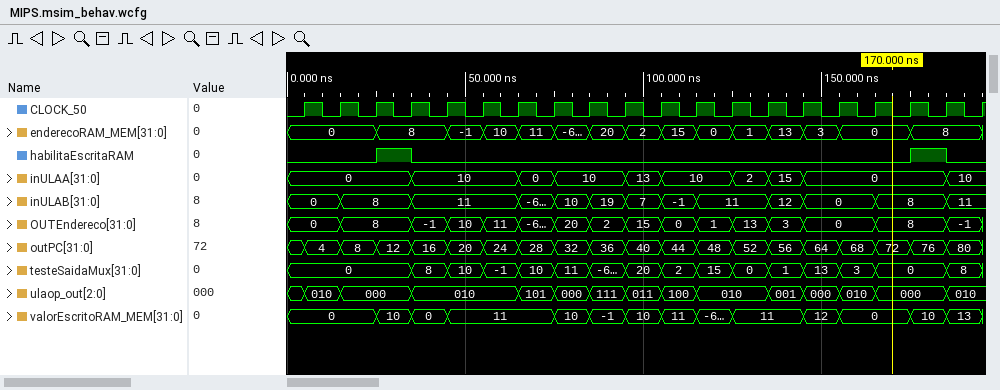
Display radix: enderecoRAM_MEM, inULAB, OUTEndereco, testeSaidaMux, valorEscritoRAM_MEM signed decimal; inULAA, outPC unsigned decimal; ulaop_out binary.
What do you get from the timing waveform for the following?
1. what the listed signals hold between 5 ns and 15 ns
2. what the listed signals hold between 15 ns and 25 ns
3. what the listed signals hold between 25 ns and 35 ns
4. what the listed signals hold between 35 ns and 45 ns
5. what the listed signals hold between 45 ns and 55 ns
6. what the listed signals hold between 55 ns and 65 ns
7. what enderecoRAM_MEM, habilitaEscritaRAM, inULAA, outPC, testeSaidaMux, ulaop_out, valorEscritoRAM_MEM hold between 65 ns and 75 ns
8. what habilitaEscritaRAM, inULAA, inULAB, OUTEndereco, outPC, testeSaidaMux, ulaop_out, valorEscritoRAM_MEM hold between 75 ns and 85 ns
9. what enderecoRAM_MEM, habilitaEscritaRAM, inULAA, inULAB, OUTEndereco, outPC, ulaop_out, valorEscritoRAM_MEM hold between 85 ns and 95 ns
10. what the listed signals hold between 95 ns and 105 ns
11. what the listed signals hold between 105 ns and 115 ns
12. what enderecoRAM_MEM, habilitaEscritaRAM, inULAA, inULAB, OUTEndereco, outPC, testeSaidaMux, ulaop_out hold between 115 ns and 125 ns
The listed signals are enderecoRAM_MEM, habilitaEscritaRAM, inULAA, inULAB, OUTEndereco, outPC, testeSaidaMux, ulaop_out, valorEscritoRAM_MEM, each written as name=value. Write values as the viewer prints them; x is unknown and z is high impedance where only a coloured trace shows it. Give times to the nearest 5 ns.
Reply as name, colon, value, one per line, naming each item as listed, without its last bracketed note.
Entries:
what the listed signals hold between 5 ns and 15 ns: enderecoRAM_MEM=0, habilitaEscritaRAM=0, inULAA=0, inULAB=0, OUTEndereco=0, outPC=4, testeSaidaMux=0, ulaop_out=010, valorEscritoRAM_MEM=0
what the listed signals hold between 15 ns and 25 ns: enderecoRAM_MEM=0, habilitaEscritaRAM=0, inULAA=0, inULAB=8, OUTEndereco=8, outPC=8, testeSaidaMux=0, ulaop_out=000, valorEscritoRAM_MEM=0
what the listed signals hold between 25 ns and 35 ns: enderecoRAM_MEM=8, habilitaEscritaRAM=1, inULAA=0, inULAB=8, OUTEndereco=8, outPC=12, testeSaidaMux=0, ulaop_out=000, valorEscritoRAM_MEM=10
what the listed signals hold between 35 ns and 45 ns: enderecoRAM_MEM=8, habilitaEscritaRAM=0, inULAA=10, inULAB=11, OUTEndereco=-1, outPC=16, testeSaidaMux=8, ulaop_out=010, valorEscritoRAM_MEM=0
what the listed signals hold between 45 ns and 55 ns: enderecoRAM_MEM=-1, habilitaEscritaRAM=0, inULAA=10, inULAB=11, OUTEndereco=10, outPC=20, testeSaidaMux=10, ulaop_out=010, valorEscritoRAM_MEM=11
what the listed signals hold between 55 ns and 65 ns: enderecoRAM_MEM=10, habilitaEscritaRAM=0, inULAA=10, inULAB=11, OUTEndereco=11, outPC=24, testeSaidaMux=-1, ulaop_out=010, valorEscritoRAM_MEM=11
what enderecoRAM_MEM, habilitaEscritaRAM, inULAA, outPC, testeSaidaMux, ulaop_out, valorEscritoRAM_MEM hold between 65 ns and 75 ns: enderecoRAM_MEM=11, habilitaEscritaRAM=0, inULAA=0, outPC=28, testeSaidaMux=10, ulaop_out=101, valorEscritoRAM_MEM=11
what habilitaEscritaRAM, inULAA, inULAB, OUTEndereco, outPC, testeSaidaMux, ulaop_out, valorEscritoRAM_MEM hold between 75 ns and 85 ns: habilitaEscritaRAM=0, inULAA=10, inULAB=10, OUTEndereco=20, outPC=32, testeSaidaMux=11, ulaop_out=000, valorEscritoRAM_MEM=10
what enderecoRAM_MEM, habilitaEscritaRAM, inULAA, inULAB, OUTEndereco, outPC, ulaop_out, valorEscritoRAM_MEM hold between 85 ns and 95 ns: enderecoRAM_MEM=20, habilitaEscritaRAM=0, inULAA=10, inULAB=19, OUTEndereco=2, outPC=36, ulaop_out=111, valorEscritoRAM_MEM=-1
what the listed signals hold between 95 ns and 105 ns: enderecoRAM_MEM=2, habilitaEscritaRAM=0, inULAA=13, inULAB=7, OUTEndereco=15, outPC=40, testeSaidaMux=20, ulaop_out=011, valorEscritoRAM_MEM=10
what the listed signals hold between 105 ns and 115 ns: enderecoRAM_MEM=15, habilitaEscritaRAM=0, inULAA=10, inULAB=-1, OUTEndereco=0, outPC=44, testeSaidaMux=2, ulaop_out=100, valorEscritoRAM_MEM=11
what enderecoRAM_MEM, habilitaEscritaRAM, inULAA, inULAB, OUTEndereco, outPC, testeSaidaMux, ulaop_out hold between 115 ns and 125 ns: enderecoRAM_MEM=0, habilitaEscritaRAM=0, inULAA=10, inULAB=11, OUTEndereco=1, outPC=48, testeSaidaMux=15, ulaop_out=010
